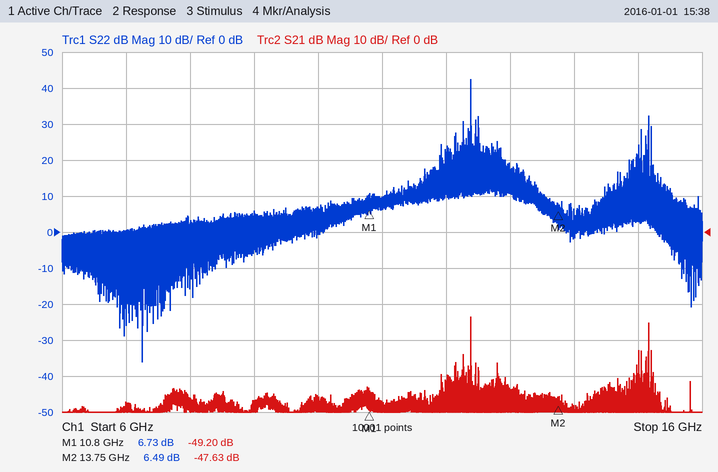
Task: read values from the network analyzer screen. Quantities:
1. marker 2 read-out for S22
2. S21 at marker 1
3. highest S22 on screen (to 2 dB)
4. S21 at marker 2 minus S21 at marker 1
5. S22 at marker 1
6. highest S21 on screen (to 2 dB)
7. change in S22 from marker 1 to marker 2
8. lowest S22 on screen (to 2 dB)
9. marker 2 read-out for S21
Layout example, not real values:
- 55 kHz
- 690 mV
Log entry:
- 6.49 dB
- -49.20 dB
- 42 dB
- 1.57 dB
- 6.73 dB
- -24 dB
- -0.24 dB
- -36 dB
- -47.63 dB
